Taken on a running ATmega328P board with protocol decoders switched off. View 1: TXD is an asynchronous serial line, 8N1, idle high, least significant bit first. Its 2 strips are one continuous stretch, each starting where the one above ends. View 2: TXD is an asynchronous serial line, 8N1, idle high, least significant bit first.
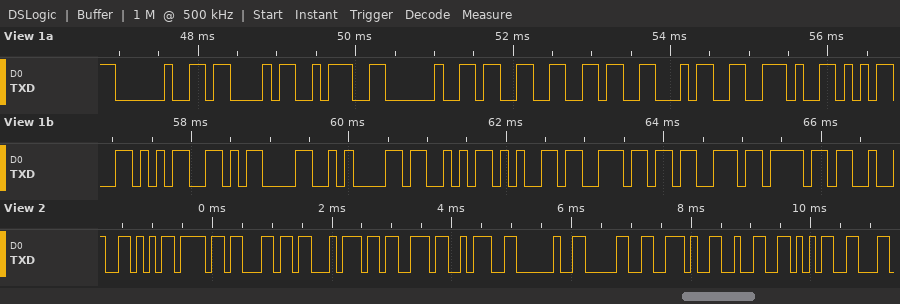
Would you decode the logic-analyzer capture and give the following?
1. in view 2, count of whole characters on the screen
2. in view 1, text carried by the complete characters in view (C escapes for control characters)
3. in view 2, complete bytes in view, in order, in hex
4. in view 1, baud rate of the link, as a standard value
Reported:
11
" C: 364.55\r\nSenso"
0x56 0x6F 0x6C 0x74 0x73 0x3A 0x20 0x30 0x2E 0x32 0x35
9600 baud
